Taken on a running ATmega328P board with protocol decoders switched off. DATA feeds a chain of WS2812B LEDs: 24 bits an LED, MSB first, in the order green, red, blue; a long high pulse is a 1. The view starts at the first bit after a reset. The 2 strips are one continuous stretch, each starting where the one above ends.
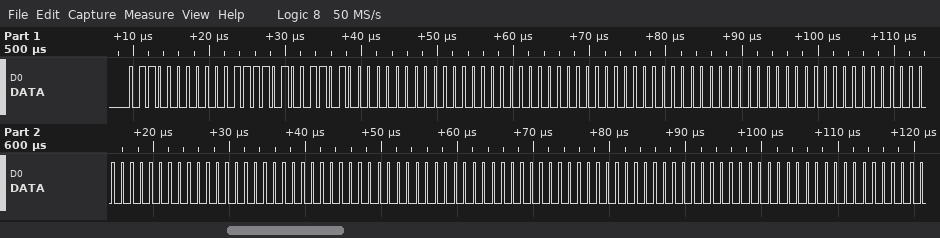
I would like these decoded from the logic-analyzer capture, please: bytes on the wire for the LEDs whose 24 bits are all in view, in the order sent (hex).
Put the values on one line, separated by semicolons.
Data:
60 1E 9A 00 00 00 00 00 00 00 00 00 00 00 00 00 00 00 00 00 00
